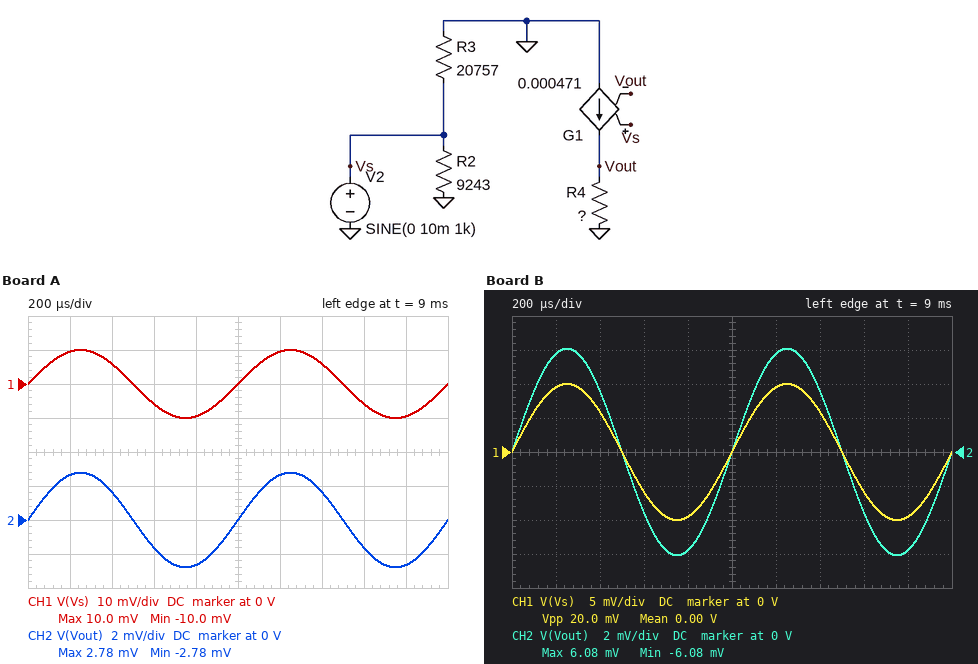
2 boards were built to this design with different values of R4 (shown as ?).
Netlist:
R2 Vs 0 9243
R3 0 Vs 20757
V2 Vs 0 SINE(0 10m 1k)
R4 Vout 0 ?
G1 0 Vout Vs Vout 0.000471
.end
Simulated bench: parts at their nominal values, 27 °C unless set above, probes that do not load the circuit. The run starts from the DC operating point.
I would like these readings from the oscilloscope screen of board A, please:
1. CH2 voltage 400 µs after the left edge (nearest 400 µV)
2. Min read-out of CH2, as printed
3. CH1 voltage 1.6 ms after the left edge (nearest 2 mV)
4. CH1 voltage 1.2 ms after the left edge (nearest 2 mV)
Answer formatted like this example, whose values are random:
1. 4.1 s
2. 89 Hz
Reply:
1. 1.6 mV
2. -2.78 mV
3. -6 mV
4. 10 mV
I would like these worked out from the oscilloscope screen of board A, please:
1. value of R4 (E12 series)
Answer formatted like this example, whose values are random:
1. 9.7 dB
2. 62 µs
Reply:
1. 820 Ω
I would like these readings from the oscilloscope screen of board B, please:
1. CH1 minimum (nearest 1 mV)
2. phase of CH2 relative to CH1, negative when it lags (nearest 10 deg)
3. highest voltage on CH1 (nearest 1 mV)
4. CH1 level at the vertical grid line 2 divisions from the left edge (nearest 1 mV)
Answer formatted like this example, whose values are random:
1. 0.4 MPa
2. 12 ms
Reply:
1. -10 mV
2. 0 deg
3. 10 mV
4. 6 mV
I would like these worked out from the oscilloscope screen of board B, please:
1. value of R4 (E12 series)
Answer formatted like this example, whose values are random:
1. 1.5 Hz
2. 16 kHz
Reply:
1. 3.3 kΩ
